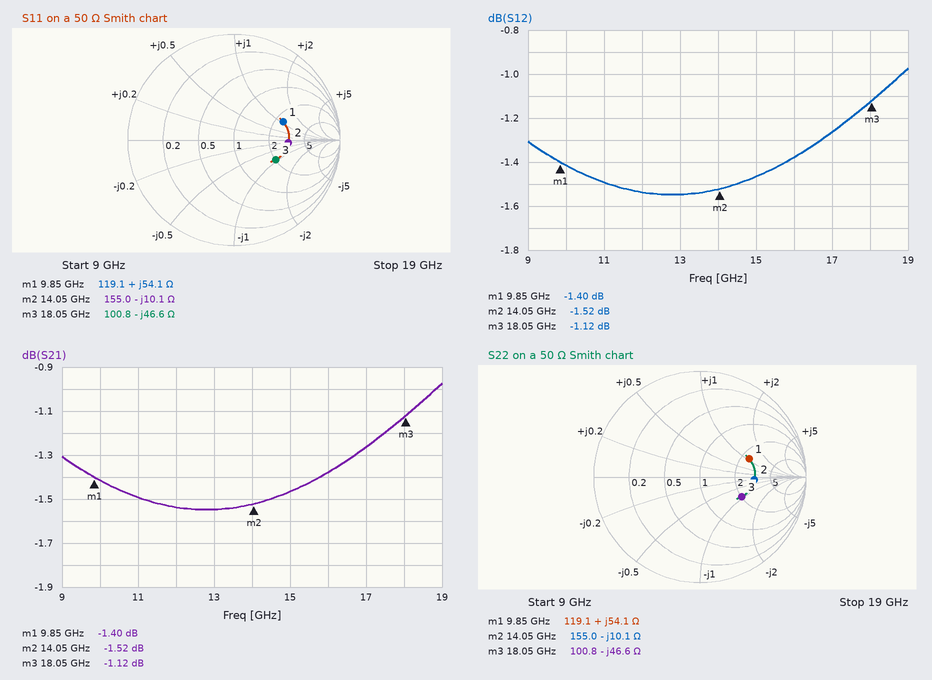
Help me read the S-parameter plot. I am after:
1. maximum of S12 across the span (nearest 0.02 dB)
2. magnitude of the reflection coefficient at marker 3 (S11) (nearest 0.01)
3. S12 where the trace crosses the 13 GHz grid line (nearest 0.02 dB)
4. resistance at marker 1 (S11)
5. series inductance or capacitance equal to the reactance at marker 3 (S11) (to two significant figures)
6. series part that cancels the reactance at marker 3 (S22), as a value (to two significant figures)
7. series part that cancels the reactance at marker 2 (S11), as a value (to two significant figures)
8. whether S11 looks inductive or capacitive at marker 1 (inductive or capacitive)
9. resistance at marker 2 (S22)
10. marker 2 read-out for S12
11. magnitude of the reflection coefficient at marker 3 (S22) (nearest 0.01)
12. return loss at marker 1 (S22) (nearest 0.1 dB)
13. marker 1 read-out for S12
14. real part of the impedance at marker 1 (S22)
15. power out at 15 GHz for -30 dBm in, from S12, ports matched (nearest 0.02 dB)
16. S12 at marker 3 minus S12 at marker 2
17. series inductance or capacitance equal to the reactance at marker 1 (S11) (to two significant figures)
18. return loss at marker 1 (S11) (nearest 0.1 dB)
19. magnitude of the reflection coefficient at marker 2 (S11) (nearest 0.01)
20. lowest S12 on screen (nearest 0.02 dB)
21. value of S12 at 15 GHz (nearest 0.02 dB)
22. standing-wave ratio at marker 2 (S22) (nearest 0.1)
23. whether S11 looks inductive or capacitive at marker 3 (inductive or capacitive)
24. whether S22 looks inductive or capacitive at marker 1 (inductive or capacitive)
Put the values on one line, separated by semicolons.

-0.98 dB; 0.44; -1.54 dB; 119.1 Ω; 190 fF; 410 pH; 110 pH; inductive; 155.0 Ω; -1.52 dB; 0.44; 6.1 dB; -1.40 dB; 119.1 Ω; -31.46 dBm; 0.40 dB; 870 pH; 6.1 dB; 0.51; -1.54 dB; -1.46 dB; 3.1; capacitive; inductive
